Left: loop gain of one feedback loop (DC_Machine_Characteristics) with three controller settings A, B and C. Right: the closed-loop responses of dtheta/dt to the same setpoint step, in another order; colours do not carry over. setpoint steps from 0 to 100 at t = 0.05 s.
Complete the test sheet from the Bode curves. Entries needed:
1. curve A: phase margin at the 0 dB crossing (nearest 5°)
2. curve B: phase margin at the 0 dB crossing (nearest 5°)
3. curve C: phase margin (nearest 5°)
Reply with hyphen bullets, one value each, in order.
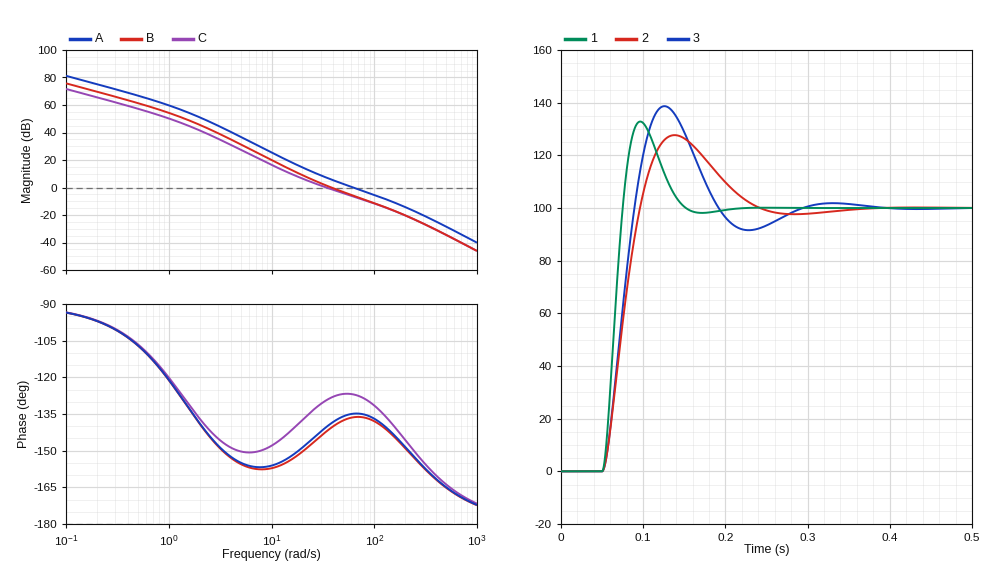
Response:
- 45°
- 40°
- 50°
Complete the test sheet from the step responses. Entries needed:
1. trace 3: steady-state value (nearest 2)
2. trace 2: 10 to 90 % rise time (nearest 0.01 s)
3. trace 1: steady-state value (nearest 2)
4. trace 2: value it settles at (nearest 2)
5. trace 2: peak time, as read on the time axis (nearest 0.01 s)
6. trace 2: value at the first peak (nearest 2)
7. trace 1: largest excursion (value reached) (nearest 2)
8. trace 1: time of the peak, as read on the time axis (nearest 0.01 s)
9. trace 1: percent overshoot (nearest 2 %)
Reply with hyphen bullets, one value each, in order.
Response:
- 100
- 0.03 s
- 100
- 100
- 0.14 s
- 128
- 132
- 0.10 s
- 32 %
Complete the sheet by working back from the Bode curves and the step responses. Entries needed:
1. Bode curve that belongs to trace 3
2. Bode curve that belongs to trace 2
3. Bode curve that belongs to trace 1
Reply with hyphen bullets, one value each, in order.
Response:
- B
- C
- A
